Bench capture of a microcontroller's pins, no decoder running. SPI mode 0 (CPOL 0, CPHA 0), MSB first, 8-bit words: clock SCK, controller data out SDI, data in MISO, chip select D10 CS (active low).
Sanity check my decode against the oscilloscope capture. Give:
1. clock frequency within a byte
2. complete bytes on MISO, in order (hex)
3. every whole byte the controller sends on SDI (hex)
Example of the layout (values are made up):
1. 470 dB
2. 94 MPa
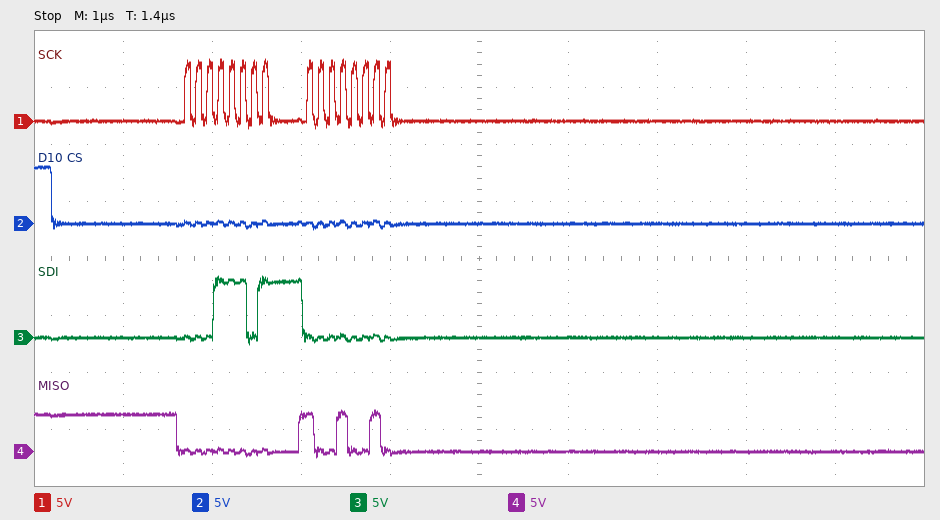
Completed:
1. 8 MHz
2. 0x00 0x92
3. 0x1D 0x00
